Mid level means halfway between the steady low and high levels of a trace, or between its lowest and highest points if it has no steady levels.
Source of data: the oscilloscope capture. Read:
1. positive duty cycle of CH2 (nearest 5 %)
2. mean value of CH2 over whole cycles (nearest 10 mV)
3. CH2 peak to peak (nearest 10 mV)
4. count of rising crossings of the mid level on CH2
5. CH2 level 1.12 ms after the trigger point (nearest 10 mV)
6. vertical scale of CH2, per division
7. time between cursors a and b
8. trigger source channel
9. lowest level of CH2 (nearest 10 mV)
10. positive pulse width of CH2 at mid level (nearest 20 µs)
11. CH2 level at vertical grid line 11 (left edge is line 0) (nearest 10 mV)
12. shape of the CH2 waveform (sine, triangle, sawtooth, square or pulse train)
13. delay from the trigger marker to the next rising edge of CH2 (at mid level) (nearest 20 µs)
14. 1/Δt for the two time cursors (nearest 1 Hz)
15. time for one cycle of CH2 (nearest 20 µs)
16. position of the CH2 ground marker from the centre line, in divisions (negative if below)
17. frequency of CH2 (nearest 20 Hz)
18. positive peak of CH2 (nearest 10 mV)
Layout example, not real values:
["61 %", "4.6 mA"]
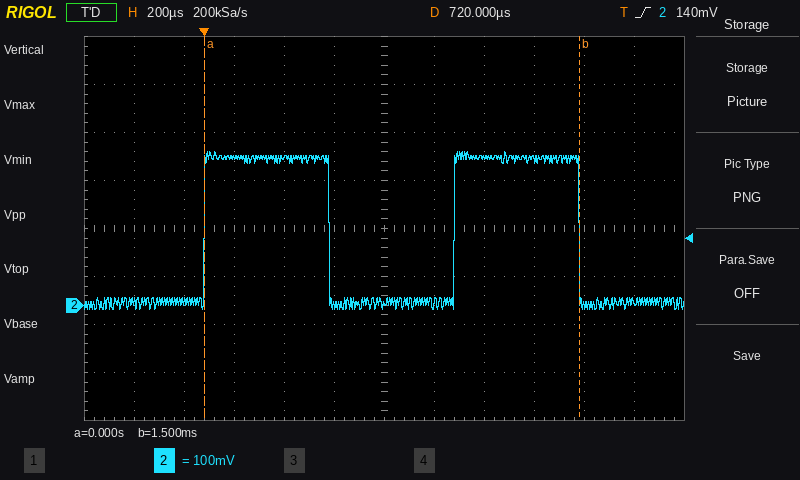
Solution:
["50 %", "160 mV", "330 mV", "2", "310 mV", "100 mV", "1.50 ms", "CH2", "-10 mV", "500 µs", "10 mV", "square", "1.00 ms", "667 Hz", "1.00 ms", "-1.6 div", "1.00 kHz", "320 mV"]
